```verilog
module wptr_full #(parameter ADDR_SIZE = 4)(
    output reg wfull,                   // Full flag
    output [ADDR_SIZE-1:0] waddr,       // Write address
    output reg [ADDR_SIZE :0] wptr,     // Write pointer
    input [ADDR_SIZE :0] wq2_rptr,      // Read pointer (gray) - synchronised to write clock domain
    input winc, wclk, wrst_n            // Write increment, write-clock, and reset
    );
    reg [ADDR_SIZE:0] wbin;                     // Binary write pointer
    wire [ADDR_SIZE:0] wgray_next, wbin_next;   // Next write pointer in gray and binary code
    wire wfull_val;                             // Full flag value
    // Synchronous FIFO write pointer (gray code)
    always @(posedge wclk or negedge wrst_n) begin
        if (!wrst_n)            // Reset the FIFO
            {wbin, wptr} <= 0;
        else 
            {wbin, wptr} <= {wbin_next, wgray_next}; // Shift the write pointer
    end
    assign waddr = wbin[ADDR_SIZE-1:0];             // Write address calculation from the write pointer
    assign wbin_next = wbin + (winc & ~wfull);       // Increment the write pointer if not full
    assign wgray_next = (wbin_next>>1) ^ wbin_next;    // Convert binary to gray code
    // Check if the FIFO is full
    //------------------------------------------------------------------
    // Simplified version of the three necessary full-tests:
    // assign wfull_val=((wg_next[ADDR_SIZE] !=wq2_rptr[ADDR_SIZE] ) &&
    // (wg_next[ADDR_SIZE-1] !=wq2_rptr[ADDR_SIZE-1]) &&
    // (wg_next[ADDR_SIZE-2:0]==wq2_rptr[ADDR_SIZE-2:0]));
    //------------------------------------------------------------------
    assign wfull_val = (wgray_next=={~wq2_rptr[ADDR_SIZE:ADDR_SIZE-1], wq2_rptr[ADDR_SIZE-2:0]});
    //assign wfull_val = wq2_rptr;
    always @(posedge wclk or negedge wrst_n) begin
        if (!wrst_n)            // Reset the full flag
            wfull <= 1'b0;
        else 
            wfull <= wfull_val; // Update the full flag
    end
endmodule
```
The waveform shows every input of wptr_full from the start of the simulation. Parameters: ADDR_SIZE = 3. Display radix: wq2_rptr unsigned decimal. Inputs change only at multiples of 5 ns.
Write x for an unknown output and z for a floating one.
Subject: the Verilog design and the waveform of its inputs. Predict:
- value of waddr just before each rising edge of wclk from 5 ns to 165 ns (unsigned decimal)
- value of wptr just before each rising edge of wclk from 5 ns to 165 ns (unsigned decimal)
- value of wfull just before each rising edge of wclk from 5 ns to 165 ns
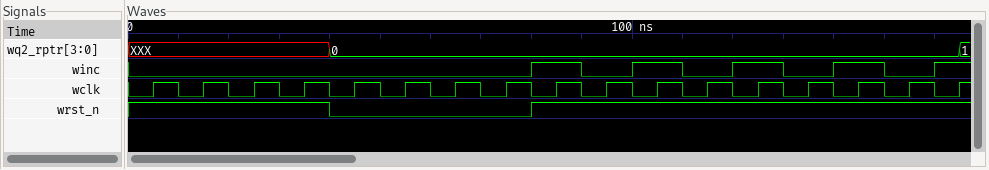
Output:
x, x, x, x, 0, 0, 0, 0, 0, 1, 1, 2, 2, 3, 3, 4, 4
x, x, x, x, 0, 0, 0, 0, 0, 1, 1, 3, 3, 2, 2, 6, 6
x x x x 0 0 0 0 0 0 0 0 0 0 0 0 0
